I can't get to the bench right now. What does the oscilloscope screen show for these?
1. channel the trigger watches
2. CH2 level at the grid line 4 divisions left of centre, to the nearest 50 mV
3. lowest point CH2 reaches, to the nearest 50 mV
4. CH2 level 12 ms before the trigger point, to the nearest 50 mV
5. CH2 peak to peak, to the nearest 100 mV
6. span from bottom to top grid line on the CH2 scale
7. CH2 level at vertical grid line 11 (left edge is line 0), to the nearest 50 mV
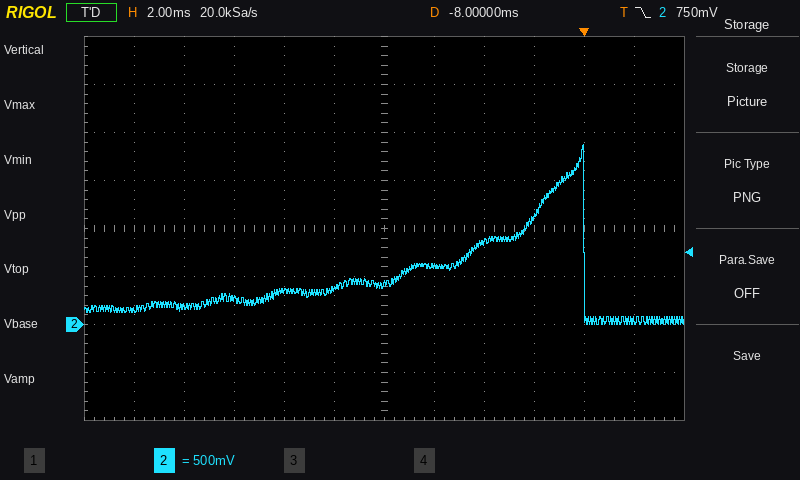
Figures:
CH2
200 mV
0 mV
350 mV
1.90 V
4 V
50 mV
